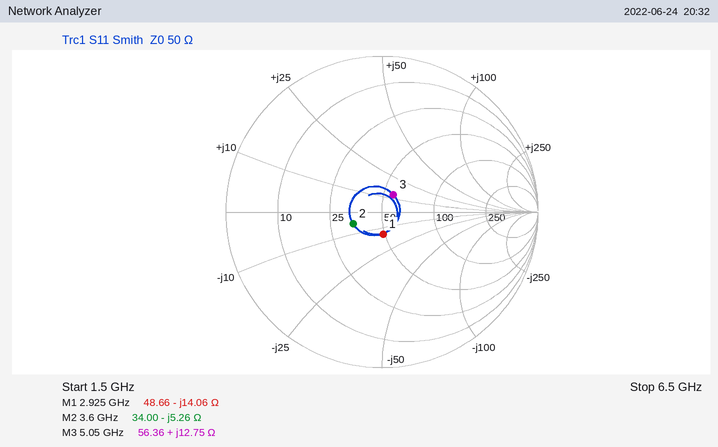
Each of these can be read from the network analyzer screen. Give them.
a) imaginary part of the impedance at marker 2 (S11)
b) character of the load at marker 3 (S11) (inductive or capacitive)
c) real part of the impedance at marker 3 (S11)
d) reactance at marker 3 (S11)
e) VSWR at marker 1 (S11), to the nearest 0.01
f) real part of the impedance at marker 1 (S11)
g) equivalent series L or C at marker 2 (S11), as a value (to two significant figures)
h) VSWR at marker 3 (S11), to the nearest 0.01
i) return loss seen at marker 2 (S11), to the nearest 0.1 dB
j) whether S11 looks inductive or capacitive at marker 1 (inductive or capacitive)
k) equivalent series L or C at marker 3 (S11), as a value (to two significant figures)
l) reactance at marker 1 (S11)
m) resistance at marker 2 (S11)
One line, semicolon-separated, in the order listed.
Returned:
-5.26 Ω; inductive; 56.36 Ω; +12.75 Ω; 1.33; 48.66 Ω; 8.4 pF; 1.31; 14.0 dB; capacitive; 400 pH; -14.06 Ω; 34.00 Ω
